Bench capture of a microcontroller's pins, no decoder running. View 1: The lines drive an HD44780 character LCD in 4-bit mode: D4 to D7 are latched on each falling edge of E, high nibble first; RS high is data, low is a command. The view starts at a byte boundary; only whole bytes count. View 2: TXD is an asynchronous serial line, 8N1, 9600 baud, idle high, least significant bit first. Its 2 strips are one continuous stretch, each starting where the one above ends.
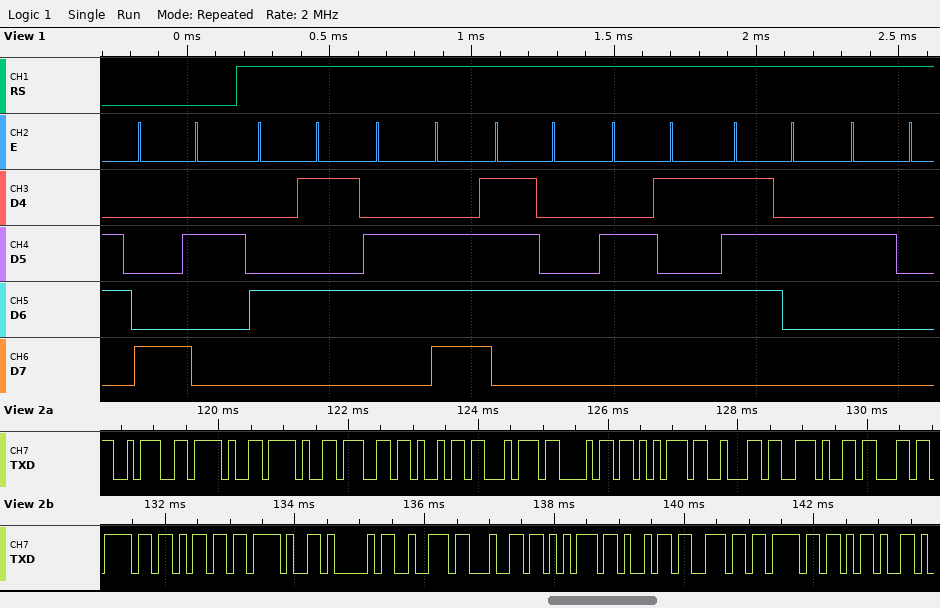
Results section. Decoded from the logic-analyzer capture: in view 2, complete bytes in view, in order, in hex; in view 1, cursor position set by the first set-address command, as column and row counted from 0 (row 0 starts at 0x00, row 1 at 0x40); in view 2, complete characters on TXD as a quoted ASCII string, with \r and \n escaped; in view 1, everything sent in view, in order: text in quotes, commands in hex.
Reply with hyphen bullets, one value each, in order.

- 3A 2F 2F 67 69 74 68 75 62 2E 63 6F 6D 2F 41 72 64 75 69 6E 6F 2D
- column 2, row 0
- "://github.com/Arduino-"
- 0x82 "Enter "
